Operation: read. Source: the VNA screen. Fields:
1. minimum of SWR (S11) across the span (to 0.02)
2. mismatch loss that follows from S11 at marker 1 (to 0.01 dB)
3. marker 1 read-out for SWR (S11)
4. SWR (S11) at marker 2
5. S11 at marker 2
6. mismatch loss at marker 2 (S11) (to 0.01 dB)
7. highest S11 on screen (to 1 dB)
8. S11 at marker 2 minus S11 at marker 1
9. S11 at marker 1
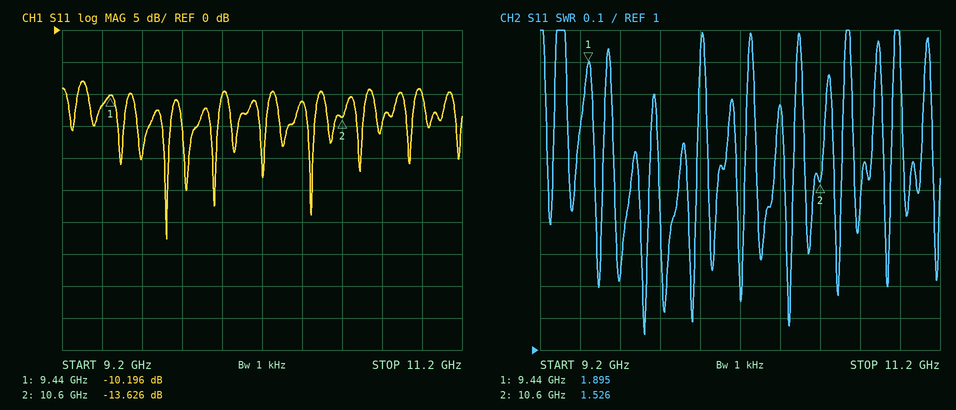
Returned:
1.04
0.44 dB
1.895
1.526
-13.626 dB
0.19 dB
-8 dB
-3.430 dB
-10.196 dB
